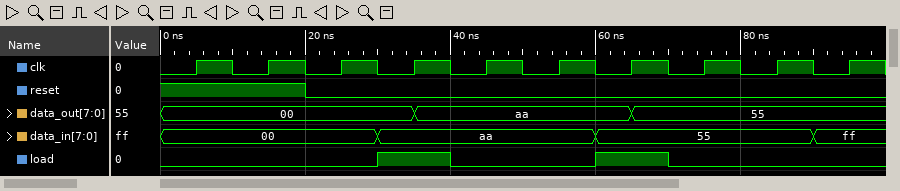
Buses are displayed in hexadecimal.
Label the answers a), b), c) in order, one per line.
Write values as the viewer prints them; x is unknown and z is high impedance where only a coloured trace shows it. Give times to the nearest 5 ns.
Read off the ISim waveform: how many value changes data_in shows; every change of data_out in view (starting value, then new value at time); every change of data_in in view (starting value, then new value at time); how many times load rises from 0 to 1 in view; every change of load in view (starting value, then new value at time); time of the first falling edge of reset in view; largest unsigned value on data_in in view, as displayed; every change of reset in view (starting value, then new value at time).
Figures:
a) 3
b) 00, aa at 35 ns, 55 at 65 ns
c) 00, aa at 30 ns, 55 at 60 ns, ff at 90 ns
d) 2
e) 0, 1 at 30 ns, 0 at 40 ns, 1 at 60 ns, 0 at 70 ns
f) 20 ns
g) ff
h) 1, 0 at 20 ns
